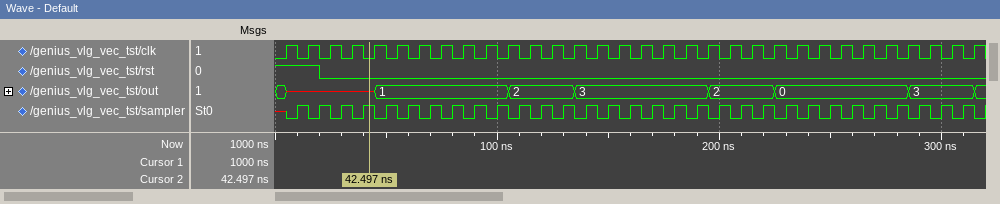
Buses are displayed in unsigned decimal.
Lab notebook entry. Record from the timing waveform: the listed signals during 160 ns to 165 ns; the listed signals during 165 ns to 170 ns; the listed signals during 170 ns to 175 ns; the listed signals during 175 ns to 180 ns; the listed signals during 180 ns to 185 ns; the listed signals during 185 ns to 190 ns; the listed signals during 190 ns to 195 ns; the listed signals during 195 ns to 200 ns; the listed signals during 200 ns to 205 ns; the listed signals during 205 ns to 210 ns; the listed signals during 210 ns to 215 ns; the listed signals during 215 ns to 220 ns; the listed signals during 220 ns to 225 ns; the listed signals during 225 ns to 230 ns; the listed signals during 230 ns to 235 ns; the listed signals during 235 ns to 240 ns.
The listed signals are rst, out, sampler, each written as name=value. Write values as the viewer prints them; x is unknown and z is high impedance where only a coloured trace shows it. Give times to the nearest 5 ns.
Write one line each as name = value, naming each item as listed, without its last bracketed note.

the listed signals during 160 ns to 165 ns = rst=0, out=3, sampler=1
the listed signals during 165 ns to 170 ns = rst=0, out=3, sampler=0
the listed signals during 170 ns to 175 ns = rst=0, out=3, sampler=1
the listed signals during 175 ns to 180 ns = rst=0, out=3, sampler=0
the listed signals during 180 ns to 185 ns = rst=0, out=3, sampler=1
the listed signals during 185 ns to 190 ns = rst=0, out=3, sampler=0
the listed signals during 190 ns to 195 ns = rst=0, out=3, sampler=1
the listed signals during 195 ns to 200 ns = rst=0, out=2, sampler=0
the listed signals during 200 ns to 205 ns = rst=0, out=2, sampler=1
the listed signals during 205 ns to 210 ns = rst=0, out=2, sampler=0
the listed signals during 210 ns to 215 ns = rst=0, out=2, sampler=1
the listed signals during 215 ns to 220 ns = rst=0, out=2, sampler=0
the listed signals during 220 ns to 225 ns = rst=0, out=2, sampler=1
the listed signals during 225 ns to 230 ns = rst=0, out=0, sampler=0
the listed signals during 230 ns to 235 ns = rst=0, out=0, sampler=1
the listed signals during 235 ns to 240 ns = rst=0, out=0, sampler=0
